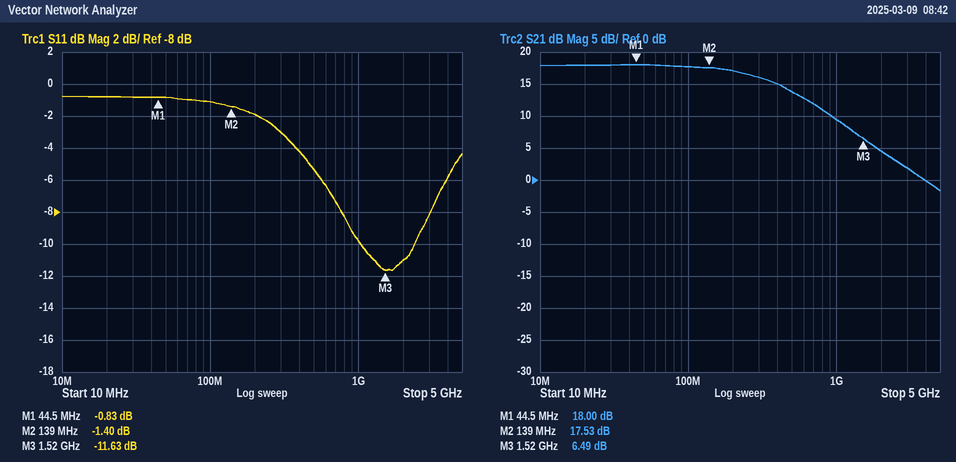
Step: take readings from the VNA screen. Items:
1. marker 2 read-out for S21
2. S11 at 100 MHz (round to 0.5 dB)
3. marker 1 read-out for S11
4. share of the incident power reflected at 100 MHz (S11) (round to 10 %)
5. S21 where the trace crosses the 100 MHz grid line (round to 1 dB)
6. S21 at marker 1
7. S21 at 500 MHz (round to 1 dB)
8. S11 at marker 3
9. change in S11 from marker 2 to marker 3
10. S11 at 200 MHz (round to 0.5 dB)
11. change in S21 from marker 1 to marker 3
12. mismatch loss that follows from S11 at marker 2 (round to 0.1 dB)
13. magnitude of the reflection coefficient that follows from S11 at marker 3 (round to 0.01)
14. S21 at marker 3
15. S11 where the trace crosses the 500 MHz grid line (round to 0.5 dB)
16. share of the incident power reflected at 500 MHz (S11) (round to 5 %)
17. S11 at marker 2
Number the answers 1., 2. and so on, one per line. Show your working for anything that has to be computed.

1. 17.53 dB
2. -1.0 dB
3. -0.83 dB
4. 10^(-1/10) ≈ 79.4 %, so 80 % to the nearest 10 %
5. 18 dB
6. 18.00 dB
7. 14 dB
8. -11.63 dB
9. -11.63 − (-1.4) = -10.23 dB
10. -2.0 dB
11. 6.49 − (18) = -11.51 dB
12. −10 log10(1 − 10^(-1.4/10)) ≈ 5.6 dB
13. 10^(-11.63/20) ≈ 0.26
14. 6.49 dB
15. -5.5 dB
16. 10^(-5.5/10) ≈ 28.2 %, so 30 % to the nearest 5 %
17. -1.40 dB
